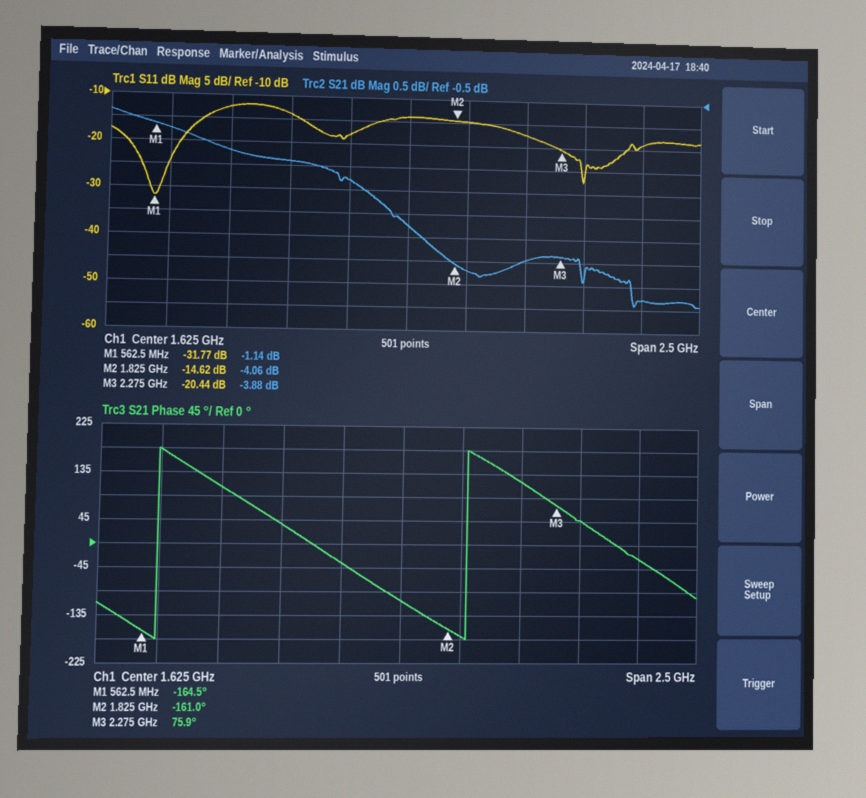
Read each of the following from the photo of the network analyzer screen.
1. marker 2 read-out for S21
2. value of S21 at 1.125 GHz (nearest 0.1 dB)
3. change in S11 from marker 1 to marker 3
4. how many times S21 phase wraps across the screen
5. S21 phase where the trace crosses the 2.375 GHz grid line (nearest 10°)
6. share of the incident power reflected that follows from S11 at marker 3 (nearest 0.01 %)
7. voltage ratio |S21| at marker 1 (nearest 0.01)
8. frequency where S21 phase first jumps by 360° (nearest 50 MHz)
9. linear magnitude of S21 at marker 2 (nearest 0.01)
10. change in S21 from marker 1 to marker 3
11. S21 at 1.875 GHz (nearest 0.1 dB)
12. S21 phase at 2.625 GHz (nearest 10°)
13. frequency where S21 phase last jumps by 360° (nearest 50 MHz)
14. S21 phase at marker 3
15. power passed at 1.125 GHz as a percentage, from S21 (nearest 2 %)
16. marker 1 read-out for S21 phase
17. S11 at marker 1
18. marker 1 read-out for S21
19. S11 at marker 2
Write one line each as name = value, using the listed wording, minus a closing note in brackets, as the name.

marker 2 read-out for S21 = -4.06 dB
value of S21 at 1.125 GHz = -1.9 dB
change in S11 from marker 1 to marker 3 = 11.33 dB
how many times S21 phase wraps across the screen = 2
S21 phase where the trace crosses the 2.375 GHz grid line = 50°
share of the incident power reflected that follows from S11 at marker 3 = 0.90 %
voltage ratio |S21| at marker 1 = 0.88
frequency where S21 phase first jumps by 360° = 600 MHz
linear magnitude of S21 at marker 2 = 0.63
change in S21 from marker 1 to marker 3 = -2.74 dB
S21 at 1.875 GHz = -4.2 dB
S21 phase at 2.625 GHz = -30°
frequency where S21 phase last jumps by 360° = 1.90 GHz
S21 phase at marker 3 = 75.9°
power passed at 1.125 GHz as a percentage, from S21 = 64 %
marker 1 read-out for S21 phase = -164.5°
S11 at marker 1 = -31.77 dB
marker 1 read-out for S21 = -1.14 dB
S11 at marker 2 = -14.62 dB
